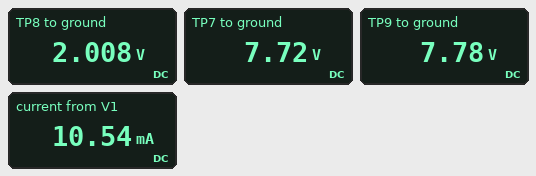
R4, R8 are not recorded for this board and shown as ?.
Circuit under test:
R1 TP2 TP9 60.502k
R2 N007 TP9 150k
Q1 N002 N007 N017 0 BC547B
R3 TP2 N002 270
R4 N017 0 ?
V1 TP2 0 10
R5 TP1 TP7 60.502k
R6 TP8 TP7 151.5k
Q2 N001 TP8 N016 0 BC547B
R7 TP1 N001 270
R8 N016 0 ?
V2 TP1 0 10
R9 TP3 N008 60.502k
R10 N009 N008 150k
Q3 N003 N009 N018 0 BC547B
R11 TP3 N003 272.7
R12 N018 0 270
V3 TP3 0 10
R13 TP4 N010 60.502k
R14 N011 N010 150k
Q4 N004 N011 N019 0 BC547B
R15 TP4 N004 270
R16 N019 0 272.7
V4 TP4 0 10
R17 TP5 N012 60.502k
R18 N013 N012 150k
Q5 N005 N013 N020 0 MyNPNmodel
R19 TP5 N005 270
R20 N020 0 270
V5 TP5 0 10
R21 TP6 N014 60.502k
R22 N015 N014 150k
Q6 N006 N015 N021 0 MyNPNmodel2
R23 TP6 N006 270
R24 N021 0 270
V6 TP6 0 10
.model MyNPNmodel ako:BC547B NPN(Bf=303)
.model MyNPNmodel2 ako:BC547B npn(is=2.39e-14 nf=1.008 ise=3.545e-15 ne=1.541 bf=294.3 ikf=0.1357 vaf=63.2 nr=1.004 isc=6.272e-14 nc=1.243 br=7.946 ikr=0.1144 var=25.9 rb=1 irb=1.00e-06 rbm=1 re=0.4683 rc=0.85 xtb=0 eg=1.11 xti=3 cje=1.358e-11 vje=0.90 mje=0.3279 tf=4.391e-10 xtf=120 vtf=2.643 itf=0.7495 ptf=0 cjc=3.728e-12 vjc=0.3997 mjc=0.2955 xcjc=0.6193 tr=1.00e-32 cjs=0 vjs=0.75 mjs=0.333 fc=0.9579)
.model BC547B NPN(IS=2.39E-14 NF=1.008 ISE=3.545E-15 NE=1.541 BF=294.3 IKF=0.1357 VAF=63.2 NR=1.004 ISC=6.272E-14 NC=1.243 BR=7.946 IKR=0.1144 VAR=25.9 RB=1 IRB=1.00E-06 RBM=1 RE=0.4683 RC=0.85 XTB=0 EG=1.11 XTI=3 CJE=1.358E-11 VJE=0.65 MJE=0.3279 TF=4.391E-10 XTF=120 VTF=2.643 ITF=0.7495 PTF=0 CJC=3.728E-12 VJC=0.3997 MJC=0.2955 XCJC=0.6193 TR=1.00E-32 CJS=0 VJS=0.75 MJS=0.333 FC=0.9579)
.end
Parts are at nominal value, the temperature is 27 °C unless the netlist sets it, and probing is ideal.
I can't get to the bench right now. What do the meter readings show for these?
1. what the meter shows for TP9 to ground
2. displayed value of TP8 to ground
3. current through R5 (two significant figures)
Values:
7.78 V
2.008 V
38 µA
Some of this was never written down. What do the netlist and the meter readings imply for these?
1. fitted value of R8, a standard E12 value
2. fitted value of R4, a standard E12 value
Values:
120 Ω
150 Ω
